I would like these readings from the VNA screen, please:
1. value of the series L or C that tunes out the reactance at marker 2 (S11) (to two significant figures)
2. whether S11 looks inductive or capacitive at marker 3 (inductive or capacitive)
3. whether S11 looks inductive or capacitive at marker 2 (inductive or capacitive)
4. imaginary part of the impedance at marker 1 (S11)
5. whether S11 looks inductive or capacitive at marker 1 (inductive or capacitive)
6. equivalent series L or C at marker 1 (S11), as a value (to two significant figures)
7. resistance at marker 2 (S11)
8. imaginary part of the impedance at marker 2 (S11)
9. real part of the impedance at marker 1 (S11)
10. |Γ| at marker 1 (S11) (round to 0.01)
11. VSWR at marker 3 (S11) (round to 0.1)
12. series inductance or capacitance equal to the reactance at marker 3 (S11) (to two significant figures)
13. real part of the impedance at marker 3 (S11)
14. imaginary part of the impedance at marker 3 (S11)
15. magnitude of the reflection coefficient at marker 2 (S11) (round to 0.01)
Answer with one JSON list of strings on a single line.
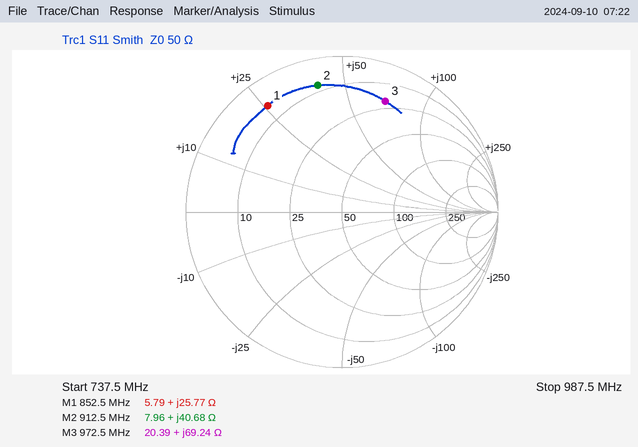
["4.3 pF", "inductive", "inductive", "+25.77 Ω", "inductive", "4.8 nH", "7.96 Ω", "+40.68 Ω", "5.79 Ω", "0.83", "7.4", "11 nH", "20.39 Ω", "+69.24 Ω", "0.83"]
